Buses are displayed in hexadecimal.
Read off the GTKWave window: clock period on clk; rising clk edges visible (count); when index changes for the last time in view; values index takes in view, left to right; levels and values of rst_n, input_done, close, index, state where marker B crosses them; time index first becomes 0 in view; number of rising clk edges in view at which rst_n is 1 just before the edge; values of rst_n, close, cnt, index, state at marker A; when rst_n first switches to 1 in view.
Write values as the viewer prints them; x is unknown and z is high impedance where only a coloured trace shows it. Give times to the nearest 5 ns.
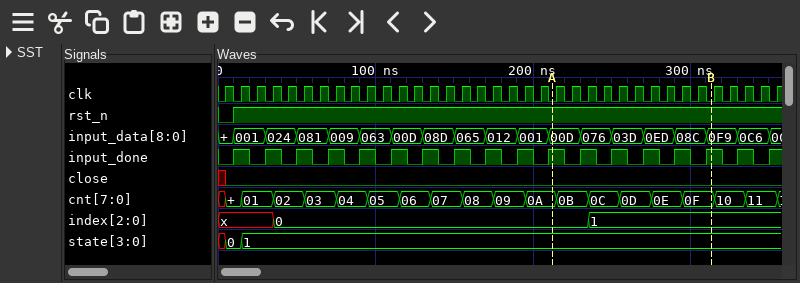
10 ns
36
235 ns
x, 0, 1
rst_n=1, input_done=1, close=0, index=1, state=1
35 ns
35
rst_n=1, close=0, cnt=0A, index=0, state=1
10 ns
